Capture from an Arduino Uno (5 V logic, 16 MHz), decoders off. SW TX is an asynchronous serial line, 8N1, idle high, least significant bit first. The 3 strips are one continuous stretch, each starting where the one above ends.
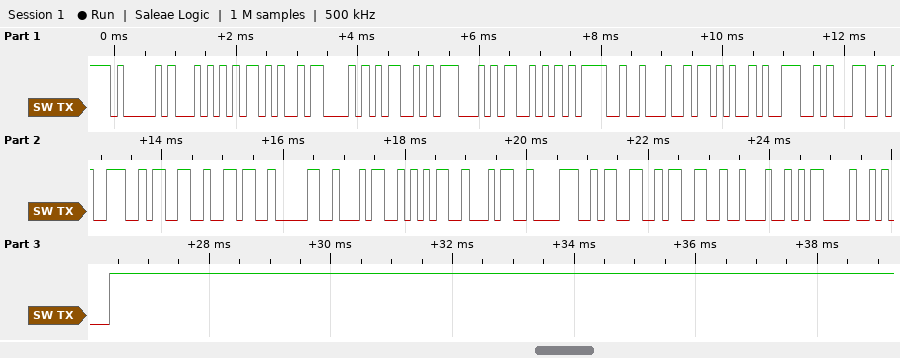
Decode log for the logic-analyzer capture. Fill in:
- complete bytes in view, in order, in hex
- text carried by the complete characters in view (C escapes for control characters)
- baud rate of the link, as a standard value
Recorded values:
41 54 2B 43 4D 47 53 3D 22 2B 39 31 39 33 36 30 34 35 34 38 33 33 22 0D 0A
"AT+CMGS=\"+919360454833\"\r\n"
9600 baud
